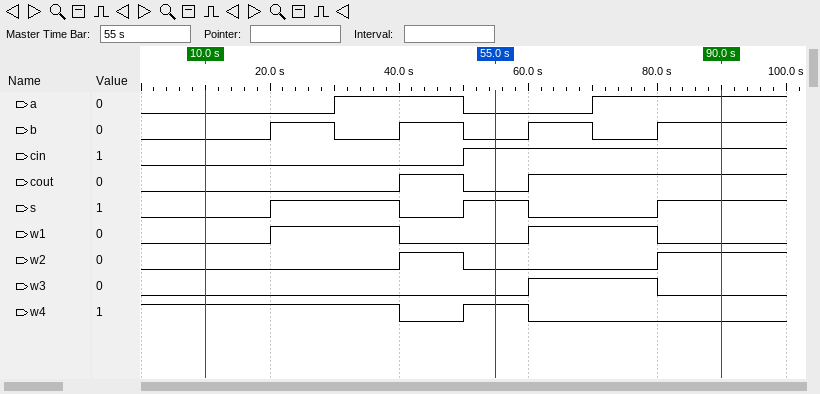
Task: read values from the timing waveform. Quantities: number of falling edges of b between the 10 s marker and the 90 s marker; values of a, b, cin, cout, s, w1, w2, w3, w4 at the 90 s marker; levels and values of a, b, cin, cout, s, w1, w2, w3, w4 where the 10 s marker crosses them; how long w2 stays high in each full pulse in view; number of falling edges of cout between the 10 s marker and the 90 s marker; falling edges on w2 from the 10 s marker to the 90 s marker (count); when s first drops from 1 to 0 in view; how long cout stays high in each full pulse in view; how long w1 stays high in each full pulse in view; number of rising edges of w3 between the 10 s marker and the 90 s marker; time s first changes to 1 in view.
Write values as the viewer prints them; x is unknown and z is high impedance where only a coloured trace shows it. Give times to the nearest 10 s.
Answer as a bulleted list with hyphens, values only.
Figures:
- 3
- a=1, b=1, cin=1, cout=1, s=1, w1=0, w2=1, w3=0, w4=0
- a=0, b=0, cin=0, cout=0, s=0, w1=0, w2=0, w3=0, w4=1
- 10 s
- 1
- 1
- 40 s
- 10 s
- 20 s, 20 s
- 1
- 20 s
